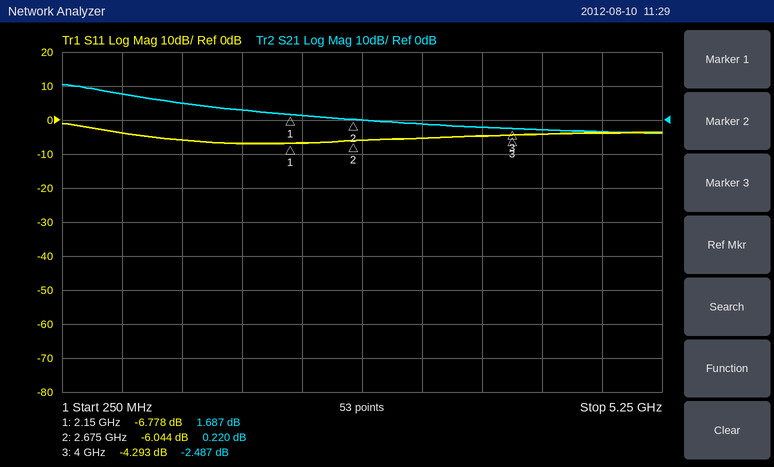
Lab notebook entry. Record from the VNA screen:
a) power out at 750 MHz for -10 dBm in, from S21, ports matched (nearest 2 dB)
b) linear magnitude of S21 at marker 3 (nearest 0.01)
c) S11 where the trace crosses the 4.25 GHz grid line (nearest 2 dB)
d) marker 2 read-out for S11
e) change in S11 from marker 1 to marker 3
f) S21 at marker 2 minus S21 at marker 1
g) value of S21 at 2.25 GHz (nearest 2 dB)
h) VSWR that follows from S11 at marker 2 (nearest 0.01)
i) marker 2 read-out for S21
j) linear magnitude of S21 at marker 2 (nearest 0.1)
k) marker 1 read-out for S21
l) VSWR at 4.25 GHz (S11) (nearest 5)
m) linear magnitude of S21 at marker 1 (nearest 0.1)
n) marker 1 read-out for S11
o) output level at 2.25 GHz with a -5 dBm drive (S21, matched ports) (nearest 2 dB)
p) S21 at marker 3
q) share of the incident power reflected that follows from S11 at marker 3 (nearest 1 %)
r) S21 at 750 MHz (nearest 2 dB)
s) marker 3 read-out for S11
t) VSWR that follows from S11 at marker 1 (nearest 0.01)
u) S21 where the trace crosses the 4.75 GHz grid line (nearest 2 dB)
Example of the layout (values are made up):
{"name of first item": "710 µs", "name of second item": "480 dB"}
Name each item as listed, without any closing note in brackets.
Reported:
{"power out at 750 MHz for -10 dBm in, from S21, ports matched": "-2 dBm", "linear magnitude of S21 at marker 3": "0.75", "S11 where the trace crosses the 4.25 GHz grid line": "-4 dB", "marker 2 read-out for S11": "-6.044 dB", "change in S11 from marker 1 to marker 3": "2.485 dB", "S21 at marker 2 minus S21 at marker 1": "-1.467 dB", "value of S21 at 2.25 GHz": "2 dB", "VSWR that follows from S11 at marker 2": "2.99", "marker 2 read-out for S21": "0.220 dB", "linear magnitude of S21 at marker 2": "1.0", "marker 1 read-out for S21": "1.687 dB", "VSWR at 4.25 GHz (S11)": "5", "linear magnitude of S21 at marker 1": "1.2", "marker 1 read-out for S11": "-6.778 dB", "output level at 2.25 GHz with a -5 dBm drive (S21, matched ports)": "-4 dBm", "S21 at marker 3": "-2.487 dB", "share of the incident power reflected that follows from S11 at marker 3": "37 %", "S21 at 750 MHz": "8 dB", "marker 3 read-out for S11": "-4.293 dB", "VSWR that follows from S11 at marker 1": "2.69", "S21 where the trace crosses the 4.75 GHz grid line": "-4 dB"}
